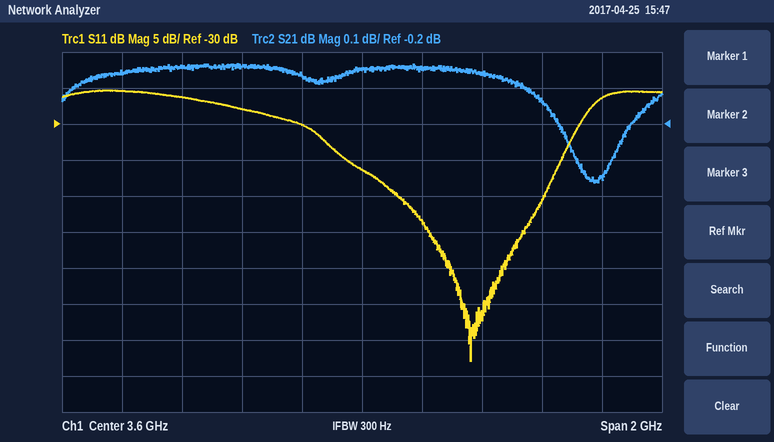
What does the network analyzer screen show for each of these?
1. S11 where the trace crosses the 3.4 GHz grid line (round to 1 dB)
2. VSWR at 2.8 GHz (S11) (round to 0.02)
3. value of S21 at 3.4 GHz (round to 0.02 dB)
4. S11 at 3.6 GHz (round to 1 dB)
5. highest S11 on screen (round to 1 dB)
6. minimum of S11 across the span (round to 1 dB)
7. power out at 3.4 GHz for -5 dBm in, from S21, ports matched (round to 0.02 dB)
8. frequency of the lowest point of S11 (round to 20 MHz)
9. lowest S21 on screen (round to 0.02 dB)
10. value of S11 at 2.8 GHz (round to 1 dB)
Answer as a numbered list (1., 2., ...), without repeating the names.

1. -30 dB
2. 1.12
3. -0.06 dB
4. -36 dB
5. -25 dB
6. -63 dB
7. -5.06 dBm
8. 3.96 GHz
9. -0.36 dB
10. -25 dB
